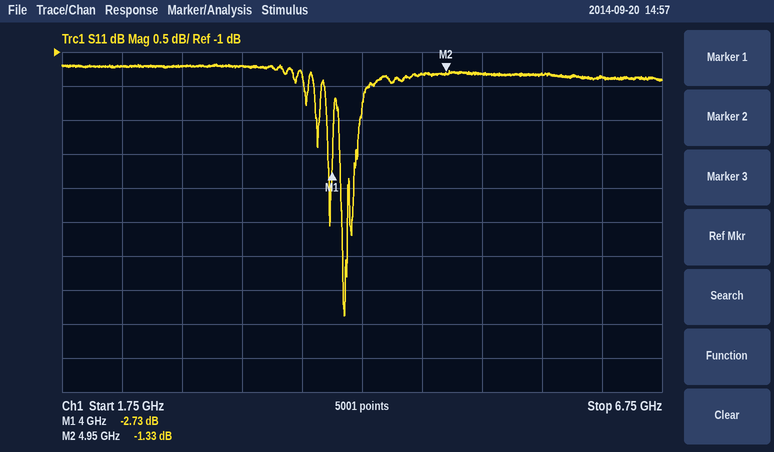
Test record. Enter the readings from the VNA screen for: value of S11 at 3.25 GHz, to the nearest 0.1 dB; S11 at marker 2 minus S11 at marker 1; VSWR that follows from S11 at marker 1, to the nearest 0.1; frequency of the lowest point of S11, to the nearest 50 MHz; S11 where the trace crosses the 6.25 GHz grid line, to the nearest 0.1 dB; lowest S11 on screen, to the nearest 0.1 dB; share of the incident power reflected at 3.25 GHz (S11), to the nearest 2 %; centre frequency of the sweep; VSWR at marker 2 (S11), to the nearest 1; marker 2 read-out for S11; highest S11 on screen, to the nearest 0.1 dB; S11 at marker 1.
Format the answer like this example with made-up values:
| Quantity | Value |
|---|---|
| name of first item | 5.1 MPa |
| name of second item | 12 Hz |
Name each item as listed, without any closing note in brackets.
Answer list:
| Quantity | Value |
|---|---|
| value of S11 at 3.25 GHz, to the nearest 0.1 dB | -1.2 dB |
| S11 at marker 2 minus S11 at marker 1 | 1.40 dB |
| VSWR that follows from S11 at marker 1, to the nearest 0.1 | 6.4 |
| frequency of the lowest point of S11, to the nearest 50 MHz | 4.10 GHz |
| S11 where the trace crosses the 6.25 GHz grid line, to the nearest 0.1 dB | -1.4 dB |
| lowest S11 on screen, to the nearest 0.1 dB | -4.9 dB |
| share of the incident power reflected at 3.25 GHz (S11), to the nearest 2 % | 76 % |
| centre frequency of the sweep | 4.25 GHz |
| VSWR at marker 2 (S11), to the nearest 1 | 13 |
| marker 2 read-out for S11 | -1.33 dB |
| highest S11 on screen, to the nearest 0.1 dB | -1.2 dB |
| S11 at marker 1 | -2.73 dB |
